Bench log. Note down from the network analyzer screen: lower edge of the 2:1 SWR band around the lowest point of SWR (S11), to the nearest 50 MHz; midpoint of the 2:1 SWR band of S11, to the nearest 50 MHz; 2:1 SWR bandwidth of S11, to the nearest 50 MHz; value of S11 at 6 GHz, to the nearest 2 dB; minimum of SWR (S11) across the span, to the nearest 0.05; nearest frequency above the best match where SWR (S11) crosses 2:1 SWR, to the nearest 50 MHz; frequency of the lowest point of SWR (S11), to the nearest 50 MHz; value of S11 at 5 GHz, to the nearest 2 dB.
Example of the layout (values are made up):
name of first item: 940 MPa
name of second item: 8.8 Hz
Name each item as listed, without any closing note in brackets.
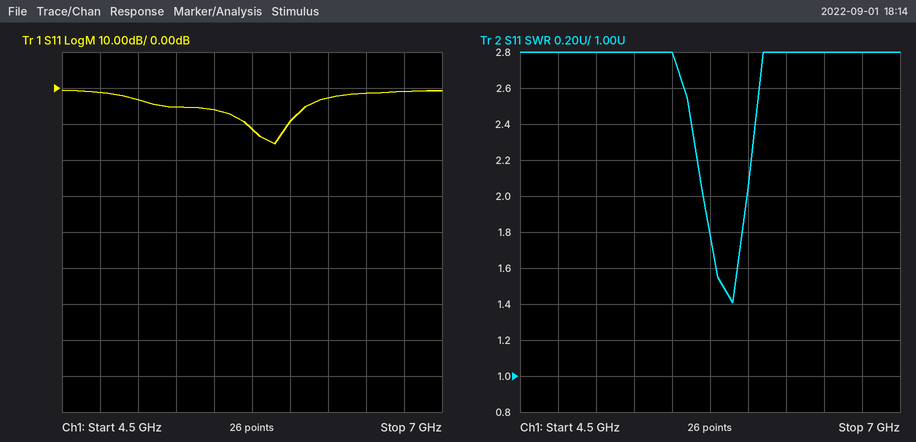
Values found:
lower edge of the 2:1 SWR band around the lowest point of SWR (S11), to the nearest 50 MHz: 5.70 GHz
midpoint of the 2:1 SWR band of S11, to the nearest 50 MHz: 5.85 GHz
2:1 SWR bandwidth of S11, to the nearest 50 MHz: 300 MHz
value of S11 at 6 GHz, to the nearest 2 dB: -10 dB
minimum of SWR (S11) across the span, to the nearest 0.05: 1.40
nearest frequency above the best match where SWR (S11) crosses 2:1 SWR, to the nearest 50 MHz: 6.00 GHz
frequency of the lowest point of SWR (S11), to the nearest 50 MHz: 5.90 GHz
value of S11 at 5 GHz, to the nearest 2 dB: -4 dB
